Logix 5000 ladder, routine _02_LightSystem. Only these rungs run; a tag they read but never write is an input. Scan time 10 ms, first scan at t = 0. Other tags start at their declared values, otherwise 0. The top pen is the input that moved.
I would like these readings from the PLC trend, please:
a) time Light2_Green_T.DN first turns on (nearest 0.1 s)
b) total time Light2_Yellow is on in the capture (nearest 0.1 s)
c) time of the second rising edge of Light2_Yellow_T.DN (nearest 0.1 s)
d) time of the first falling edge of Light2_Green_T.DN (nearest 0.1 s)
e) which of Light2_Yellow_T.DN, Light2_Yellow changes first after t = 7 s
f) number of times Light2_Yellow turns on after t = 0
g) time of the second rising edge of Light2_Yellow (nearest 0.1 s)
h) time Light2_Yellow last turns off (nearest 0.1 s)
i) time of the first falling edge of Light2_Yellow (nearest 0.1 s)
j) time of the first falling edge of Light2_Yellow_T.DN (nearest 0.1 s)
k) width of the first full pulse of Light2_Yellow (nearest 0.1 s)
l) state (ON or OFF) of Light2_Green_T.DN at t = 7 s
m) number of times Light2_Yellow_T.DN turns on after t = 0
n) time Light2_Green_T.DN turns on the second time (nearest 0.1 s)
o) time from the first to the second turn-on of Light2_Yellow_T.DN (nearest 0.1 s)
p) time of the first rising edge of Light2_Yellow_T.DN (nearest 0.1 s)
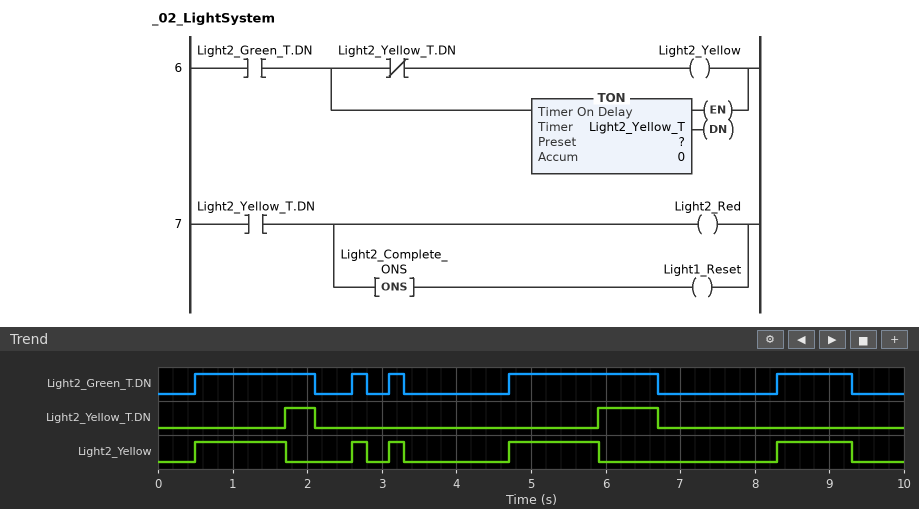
0.5 s
3.8 s
5.9 s
2.1 s
Light2_Yellow
5
2.6 s
9.3 s
1.7 s
2.1 s
1.2 s
OFF
2
2.6 s
4.2 s
1.7 s
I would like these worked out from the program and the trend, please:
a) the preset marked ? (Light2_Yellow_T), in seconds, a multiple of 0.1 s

1.2 s
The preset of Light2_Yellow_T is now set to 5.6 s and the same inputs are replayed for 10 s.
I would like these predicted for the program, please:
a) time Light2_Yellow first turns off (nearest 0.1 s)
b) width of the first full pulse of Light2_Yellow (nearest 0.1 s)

2.1 s
1.6 s
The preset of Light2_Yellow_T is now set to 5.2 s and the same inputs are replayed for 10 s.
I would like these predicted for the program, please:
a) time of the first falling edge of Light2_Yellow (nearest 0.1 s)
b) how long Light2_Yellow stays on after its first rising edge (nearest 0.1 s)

2.1 s
1.6 s
